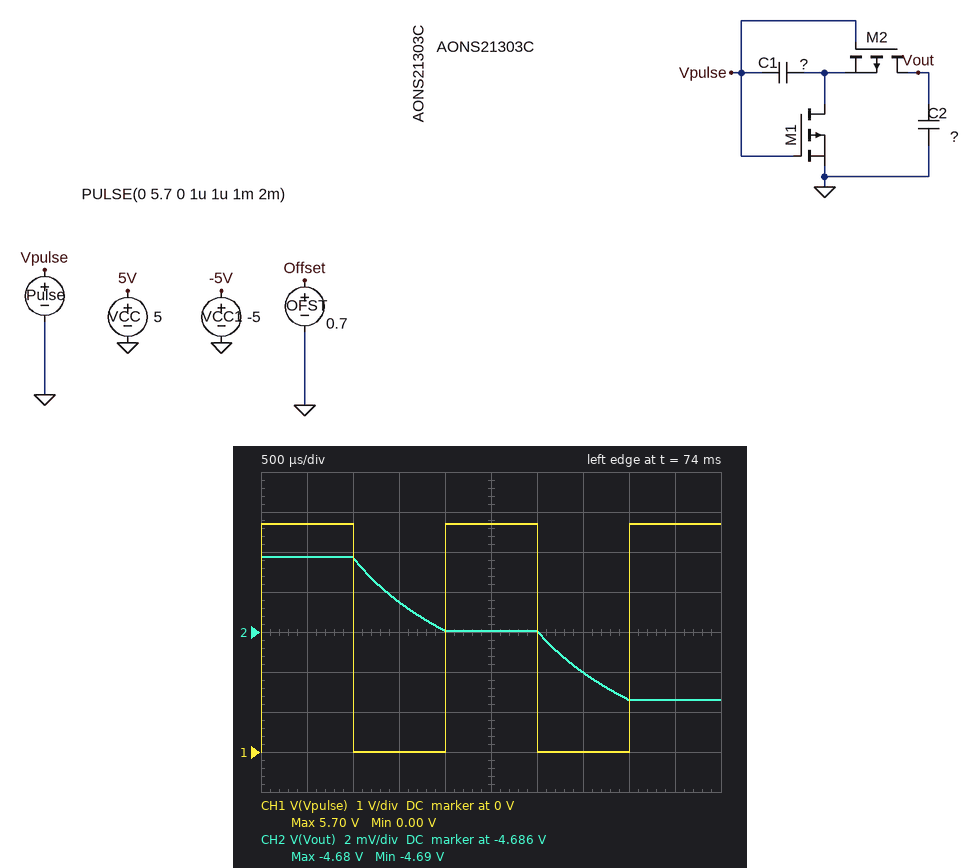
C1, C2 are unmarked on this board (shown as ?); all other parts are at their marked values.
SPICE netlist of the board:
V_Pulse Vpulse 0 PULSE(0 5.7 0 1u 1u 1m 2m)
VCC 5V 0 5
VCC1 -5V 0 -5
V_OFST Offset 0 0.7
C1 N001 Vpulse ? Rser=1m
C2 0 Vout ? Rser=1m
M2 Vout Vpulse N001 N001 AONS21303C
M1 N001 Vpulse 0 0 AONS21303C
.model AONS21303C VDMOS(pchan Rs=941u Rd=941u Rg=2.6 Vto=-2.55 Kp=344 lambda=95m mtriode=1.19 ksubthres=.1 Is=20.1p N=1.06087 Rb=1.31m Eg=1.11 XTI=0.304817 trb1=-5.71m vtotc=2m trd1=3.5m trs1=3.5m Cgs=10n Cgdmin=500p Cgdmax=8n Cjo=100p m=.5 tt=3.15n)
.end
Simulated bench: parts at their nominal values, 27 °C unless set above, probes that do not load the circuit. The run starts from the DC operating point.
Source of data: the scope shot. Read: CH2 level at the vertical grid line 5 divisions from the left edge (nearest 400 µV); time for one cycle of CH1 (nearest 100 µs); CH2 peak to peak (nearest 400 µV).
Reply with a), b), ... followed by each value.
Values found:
a) -4.6860 V
b) 2.0 ms
c) 7.2 mV
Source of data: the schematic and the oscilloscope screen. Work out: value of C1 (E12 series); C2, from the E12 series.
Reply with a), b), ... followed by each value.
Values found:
a) 100 µF
b) 560 µF
